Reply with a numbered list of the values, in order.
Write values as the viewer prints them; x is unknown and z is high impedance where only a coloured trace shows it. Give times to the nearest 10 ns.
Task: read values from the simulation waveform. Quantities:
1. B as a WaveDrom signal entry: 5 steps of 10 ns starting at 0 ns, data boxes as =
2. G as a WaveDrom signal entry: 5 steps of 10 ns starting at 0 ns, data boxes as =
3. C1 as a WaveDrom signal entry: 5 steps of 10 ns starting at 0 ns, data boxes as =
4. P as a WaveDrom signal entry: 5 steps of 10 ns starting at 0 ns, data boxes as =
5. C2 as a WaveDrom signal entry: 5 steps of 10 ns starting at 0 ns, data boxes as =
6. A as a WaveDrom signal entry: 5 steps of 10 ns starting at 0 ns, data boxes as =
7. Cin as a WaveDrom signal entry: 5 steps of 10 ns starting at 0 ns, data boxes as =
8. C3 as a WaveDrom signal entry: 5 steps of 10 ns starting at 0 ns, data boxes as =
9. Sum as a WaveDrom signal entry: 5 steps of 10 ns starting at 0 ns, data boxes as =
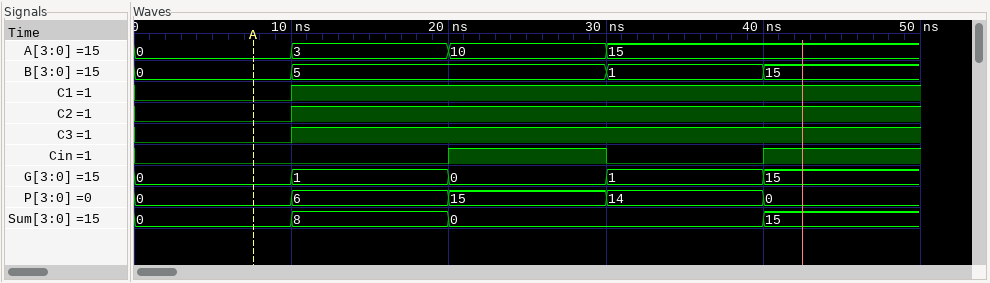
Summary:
1. {name: 'B', wave: '==.==', data: '0 5 1 15'}
2. {name: 'G', wave: '=====', data: '0 1 0 1 15'}
3. {name: 'C1', wave: '01...'}
4. {name: 'P', wave: '=====', data: '0 6 15 14 0'}
5. {name: 'C2', wave: '01...'}
6. {name: 'A', wave: '====.', data: '0 3 10 15'}
7. {name: 'Cin', wave: '0.101'}
8. {name: 'C3', wave: '01...'}
9. {name: 'Sum', wave: '===.=', data: '0 8 0 15'}
